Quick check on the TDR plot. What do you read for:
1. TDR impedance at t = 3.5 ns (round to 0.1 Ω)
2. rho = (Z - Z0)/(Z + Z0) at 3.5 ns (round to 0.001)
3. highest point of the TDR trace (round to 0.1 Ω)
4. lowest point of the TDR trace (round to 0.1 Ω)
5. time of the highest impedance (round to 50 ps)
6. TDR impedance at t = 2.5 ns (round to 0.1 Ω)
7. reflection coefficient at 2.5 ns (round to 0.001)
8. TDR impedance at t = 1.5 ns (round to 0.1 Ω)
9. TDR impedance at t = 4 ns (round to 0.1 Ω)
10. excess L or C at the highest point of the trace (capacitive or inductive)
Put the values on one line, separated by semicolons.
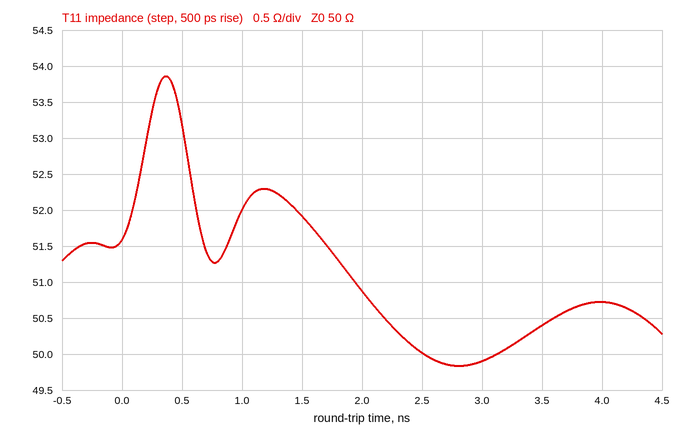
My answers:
50.4 Ω; +0.004; 53.9 Ω; 49.8 Ω; 350 ps; 50.0 Ω; 0.000; 51.9 Ω; 50.7 Ω; inductive
